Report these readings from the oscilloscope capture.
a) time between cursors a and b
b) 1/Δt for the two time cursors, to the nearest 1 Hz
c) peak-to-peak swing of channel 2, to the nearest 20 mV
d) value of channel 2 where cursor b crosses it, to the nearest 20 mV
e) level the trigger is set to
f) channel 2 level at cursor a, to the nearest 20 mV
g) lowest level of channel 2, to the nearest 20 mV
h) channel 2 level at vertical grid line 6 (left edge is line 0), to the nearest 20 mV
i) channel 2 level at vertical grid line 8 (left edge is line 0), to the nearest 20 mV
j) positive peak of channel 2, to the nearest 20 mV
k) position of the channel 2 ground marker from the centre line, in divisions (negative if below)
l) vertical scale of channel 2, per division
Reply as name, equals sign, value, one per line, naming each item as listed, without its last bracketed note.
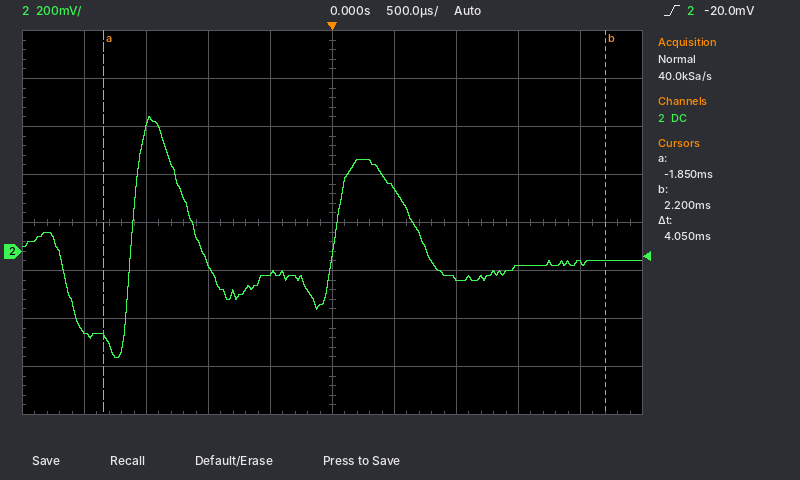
time between cursors a and b = 4.05 ms
1/Δt for the two time cursors, to the nearest 1 Hz = 247 Hz
peak-to-peak swing of channel 2, to the nearest 20 mV = 1.00 V
value of channel 2 where cursor b crosses it, to the nearest 20 mV = -40 mV
level the trigger is set to = -20.0 mV
channel 2 level at cursor a, to the nearest 20 mV = -360 mV
lowest level of channel 2, to the nearest 20 mV = -440 mV
channel 2 level at vertical grid line 6 (left edge is line 0), to the nearest 20 mV = 260 mV
channel 2 level at vertical grid line 8 (left edge is line 0), to the nearest 20 mV = -60 mV
positive peak of channel 2, to the nearest 20 mV = 560 mV
position of the channel 2 ground marker from the centre line, in divisions = -0.6 div
vertical scale of channel 2, per division = 200 mV
